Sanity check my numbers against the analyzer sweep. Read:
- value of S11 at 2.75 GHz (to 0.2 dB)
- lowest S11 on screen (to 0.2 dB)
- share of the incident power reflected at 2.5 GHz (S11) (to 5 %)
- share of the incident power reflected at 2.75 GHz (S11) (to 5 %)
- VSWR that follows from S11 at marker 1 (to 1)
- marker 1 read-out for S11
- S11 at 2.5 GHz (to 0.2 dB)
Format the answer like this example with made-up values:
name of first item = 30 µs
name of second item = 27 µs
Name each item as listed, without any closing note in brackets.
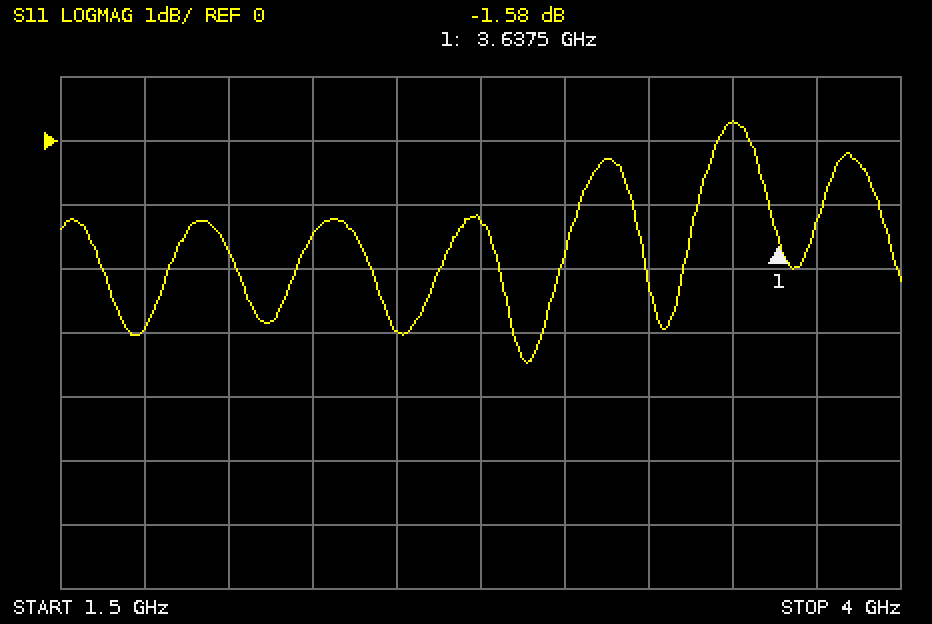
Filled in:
value of S11 at 2.75 GHz = -1.2 dB
lowest S11 on screen = -3.4 dB
share of the incident power reflected at 2.5 GHz (S11) = 50 %
share of the incident power reflected at 2.75 GHz (S11) = 75 %
VSWR that follows from S11 at marker 1 = 11
marker 1 read-out for S11 = -1.58 dB
S11 at 2.5 GHz = -3.0 dB
